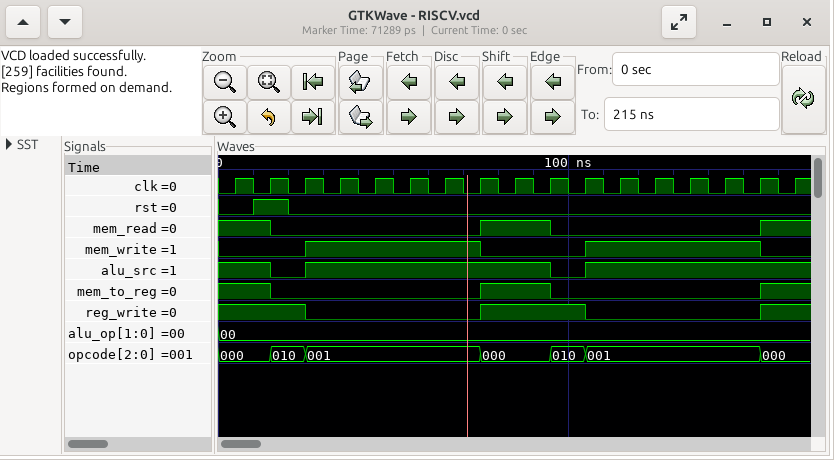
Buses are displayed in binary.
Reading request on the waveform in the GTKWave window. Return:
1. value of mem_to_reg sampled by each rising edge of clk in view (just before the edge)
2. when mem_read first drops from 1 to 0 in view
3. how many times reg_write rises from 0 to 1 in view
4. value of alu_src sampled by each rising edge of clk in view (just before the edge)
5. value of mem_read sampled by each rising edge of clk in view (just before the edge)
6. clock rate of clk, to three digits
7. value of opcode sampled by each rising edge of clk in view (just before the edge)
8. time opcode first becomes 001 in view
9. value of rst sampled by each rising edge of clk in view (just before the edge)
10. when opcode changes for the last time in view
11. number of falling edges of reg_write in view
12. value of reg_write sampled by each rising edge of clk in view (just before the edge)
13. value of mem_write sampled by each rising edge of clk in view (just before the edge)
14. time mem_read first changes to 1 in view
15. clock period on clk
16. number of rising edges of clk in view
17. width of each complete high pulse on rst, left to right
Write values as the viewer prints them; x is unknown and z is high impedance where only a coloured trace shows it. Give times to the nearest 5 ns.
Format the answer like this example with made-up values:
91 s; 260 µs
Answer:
1 1 0 0 0 0 0 0 1 1 0 0 0 0 0 0 1; 15 ns; 2; 1 1 0 1 1 1 1 1 1 1 0 1 1 1 1 1 1; 1 1 0 0 0 0 0 0 1 1 0 0 0 0 0 0 1; 100 MHz; 000, 000, 010, 001, 001, 001, 001, 001, 000, 000, 010, 001, 001, 001, 001, 001, 000; 25 ns; 0 1 0 0 0 0 0 0 0 0 0 0 0 0 0 0 0; 155 ns; 2; 1 1 1 0 0 0 0 0 1 1 1 0 0 0 0 0 1; 0 0 0 1 1 1 1 1 0 0 0 1 1 1 1 1 0; 75 ns; 10 ns; 17; 10 ns
